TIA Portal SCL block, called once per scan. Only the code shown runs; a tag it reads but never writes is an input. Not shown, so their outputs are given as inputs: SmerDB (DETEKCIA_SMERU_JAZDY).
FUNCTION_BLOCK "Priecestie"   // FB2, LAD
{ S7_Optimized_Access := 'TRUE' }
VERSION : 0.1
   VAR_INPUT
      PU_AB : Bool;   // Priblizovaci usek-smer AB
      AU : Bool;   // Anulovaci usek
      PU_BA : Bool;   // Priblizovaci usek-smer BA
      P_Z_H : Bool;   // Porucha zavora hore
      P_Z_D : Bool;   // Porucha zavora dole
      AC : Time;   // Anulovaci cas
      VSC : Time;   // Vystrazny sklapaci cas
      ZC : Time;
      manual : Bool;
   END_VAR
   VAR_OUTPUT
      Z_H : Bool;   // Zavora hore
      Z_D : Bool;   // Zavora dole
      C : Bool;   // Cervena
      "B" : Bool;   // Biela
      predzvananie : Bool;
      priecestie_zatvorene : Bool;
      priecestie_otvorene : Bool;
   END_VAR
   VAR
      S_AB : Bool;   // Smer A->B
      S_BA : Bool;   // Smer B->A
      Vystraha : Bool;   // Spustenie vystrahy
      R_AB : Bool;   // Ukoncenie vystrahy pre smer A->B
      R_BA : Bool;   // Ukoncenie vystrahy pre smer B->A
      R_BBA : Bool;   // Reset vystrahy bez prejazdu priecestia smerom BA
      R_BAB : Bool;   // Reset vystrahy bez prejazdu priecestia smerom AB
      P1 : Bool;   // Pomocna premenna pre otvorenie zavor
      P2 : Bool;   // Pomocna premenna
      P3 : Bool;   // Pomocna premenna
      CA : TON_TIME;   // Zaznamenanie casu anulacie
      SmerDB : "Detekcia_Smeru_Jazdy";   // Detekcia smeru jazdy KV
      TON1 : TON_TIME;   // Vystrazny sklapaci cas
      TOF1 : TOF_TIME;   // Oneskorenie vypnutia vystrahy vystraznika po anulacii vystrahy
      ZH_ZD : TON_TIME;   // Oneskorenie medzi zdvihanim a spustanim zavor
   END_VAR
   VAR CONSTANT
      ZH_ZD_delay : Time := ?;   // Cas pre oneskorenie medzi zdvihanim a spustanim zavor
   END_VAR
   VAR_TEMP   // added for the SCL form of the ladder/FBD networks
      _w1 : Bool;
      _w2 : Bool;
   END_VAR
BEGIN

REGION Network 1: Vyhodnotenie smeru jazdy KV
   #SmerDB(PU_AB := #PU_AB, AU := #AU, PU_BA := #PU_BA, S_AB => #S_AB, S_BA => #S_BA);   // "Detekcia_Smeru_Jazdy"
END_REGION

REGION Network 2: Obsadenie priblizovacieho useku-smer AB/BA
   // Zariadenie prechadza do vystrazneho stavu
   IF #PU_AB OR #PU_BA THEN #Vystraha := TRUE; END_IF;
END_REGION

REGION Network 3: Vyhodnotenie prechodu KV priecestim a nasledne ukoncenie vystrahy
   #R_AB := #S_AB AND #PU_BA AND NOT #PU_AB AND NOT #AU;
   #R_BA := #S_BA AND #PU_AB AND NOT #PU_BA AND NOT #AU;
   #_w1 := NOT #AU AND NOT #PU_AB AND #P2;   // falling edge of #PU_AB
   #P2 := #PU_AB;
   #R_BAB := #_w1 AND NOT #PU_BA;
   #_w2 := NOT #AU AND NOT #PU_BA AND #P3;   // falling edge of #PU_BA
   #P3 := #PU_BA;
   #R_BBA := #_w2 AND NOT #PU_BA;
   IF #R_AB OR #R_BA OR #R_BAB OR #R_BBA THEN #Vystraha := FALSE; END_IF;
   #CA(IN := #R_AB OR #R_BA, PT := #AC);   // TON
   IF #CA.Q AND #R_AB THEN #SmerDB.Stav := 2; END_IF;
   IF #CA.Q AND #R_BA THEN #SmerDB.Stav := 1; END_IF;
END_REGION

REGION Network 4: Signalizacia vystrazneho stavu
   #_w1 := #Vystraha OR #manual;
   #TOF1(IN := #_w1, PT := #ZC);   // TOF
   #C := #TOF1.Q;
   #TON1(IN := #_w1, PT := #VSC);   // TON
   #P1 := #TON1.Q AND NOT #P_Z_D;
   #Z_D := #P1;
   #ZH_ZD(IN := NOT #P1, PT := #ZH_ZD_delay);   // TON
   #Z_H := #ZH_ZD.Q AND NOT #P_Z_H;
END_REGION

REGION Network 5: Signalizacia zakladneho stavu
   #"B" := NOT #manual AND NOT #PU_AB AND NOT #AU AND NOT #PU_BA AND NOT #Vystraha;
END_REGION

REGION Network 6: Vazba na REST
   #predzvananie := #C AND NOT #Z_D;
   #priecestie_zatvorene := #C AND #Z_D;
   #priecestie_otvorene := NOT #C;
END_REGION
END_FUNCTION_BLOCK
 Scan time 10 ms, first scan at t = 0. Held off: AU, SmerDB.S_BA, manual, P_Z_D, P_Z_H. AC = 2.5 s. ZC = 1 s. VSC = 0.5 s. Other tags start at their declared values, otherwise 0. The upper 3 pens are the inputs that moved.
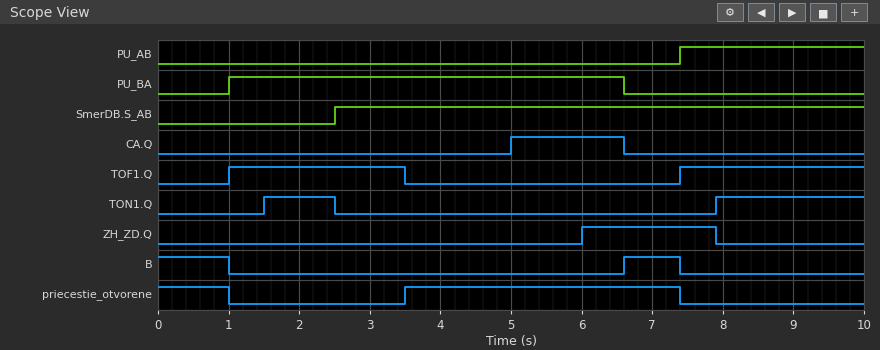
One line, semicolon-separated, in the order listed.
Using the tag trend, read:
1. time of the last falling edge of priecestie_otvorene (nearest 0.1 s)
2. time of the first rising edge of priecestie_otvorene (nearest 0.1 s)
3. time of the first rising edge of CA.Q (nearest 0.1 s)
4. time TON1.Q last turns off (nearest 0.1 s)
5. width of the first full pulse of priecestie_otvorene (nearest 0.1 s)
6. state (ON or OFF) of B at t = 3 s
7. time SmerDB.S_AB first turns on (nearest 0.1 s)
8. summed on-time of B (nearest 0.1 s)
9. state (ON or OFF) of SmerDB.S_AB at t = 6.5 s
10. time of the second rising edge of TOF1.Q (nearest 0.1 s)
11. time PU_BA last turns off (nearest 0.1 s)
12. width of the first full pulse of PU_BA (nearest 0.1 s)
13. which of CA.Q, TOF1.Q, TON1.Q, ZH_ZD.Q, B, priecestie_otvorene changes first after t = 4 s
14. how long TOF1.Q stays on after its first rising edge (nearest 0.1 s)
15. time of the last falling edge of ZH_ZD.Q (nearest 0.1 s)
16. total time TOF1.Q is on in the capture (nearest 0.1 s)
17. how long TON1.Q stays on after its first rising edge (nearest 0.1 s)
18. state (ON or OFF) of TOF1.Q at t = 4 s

7.4 s; 3.5 s; 5.0 s; 2.5 s; 3.9 s; OFF; 2.5 s; 1.8 s; ON; 7.4 s; 6.6 s; 5.6 s; CA.Q; 2.5 s; 7.9 s; 5.1 s; 1.0 s; OFF
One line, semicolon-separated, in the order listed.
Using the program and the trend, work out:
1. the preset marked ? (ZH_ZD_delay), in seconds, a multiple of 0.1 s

3.5 s
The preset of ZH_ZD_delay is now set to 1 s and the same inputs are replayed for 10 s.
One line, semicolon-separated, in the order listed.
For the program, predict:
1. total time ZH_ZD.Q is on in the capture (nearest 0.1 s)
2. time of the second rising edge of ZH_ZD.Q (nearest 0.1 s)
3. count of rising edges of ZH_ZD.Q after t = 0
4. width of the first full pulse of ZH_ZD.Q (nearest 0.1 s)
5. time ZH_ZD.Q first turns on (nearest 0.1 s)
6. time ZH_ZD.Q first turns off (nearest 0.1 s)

4.9 s; 3.5 s; 2; 0.5 s; 1.0 s; 1.5 s
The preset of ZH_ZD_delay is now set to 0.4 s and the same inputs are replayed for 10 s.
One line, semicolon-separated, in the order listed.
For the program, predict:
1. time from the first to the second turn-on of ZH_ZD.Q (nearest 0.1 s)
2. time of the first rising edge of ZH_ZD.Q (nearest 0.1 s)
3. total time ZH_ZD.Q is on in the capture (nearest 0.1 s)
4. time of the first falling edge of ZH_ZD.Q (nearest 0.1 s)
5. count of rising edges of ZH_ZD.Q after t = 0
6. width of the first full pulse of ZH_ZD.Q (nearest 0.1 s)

2.5 s; 0.4 s; 6.1 s; 1.5 s; 2; 1.1 s
